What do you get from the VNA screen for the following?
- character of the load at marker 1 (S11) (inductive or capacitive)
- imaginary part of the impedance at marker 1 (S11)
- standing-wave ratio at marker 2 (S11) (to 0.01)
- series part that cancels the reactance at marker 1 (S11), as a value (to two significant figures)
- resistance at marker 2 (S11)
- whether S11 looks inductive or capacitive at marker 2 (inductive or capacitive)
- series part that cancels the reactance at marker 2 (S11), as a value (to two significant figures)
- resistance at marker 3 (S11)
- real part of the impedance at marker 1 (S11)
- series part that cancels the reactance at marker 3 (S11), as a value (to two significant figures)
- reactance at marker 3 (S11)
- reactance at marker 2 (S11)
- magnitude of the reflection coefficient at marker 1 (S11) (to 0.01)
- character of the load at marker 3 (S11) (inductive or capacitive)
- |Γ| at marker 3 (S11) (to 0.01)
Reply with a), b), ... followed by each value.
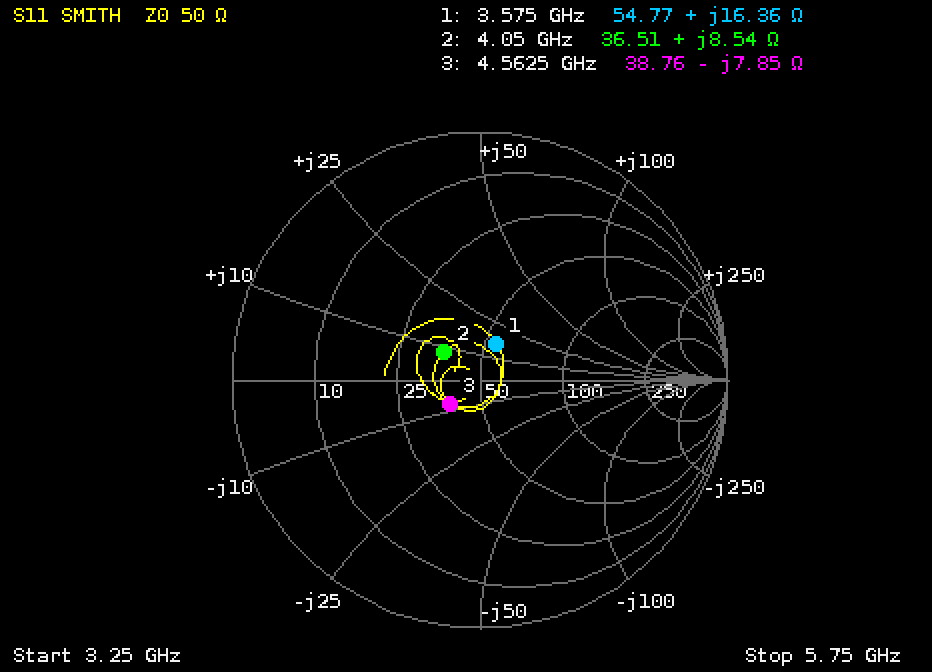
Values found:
a) inductive
b) +16.36 Ω
c) 1.45
d) 2.7 pF
e) 36.51 Ω
f) inductive
g) 4.6 pF
h) 38.76 Ω
i) 54.77 Ω
j) 270 pH
k) -7.85 Ω
l) +8.54 Ω
m) 0.16
n) capacitive
o) 0.15
